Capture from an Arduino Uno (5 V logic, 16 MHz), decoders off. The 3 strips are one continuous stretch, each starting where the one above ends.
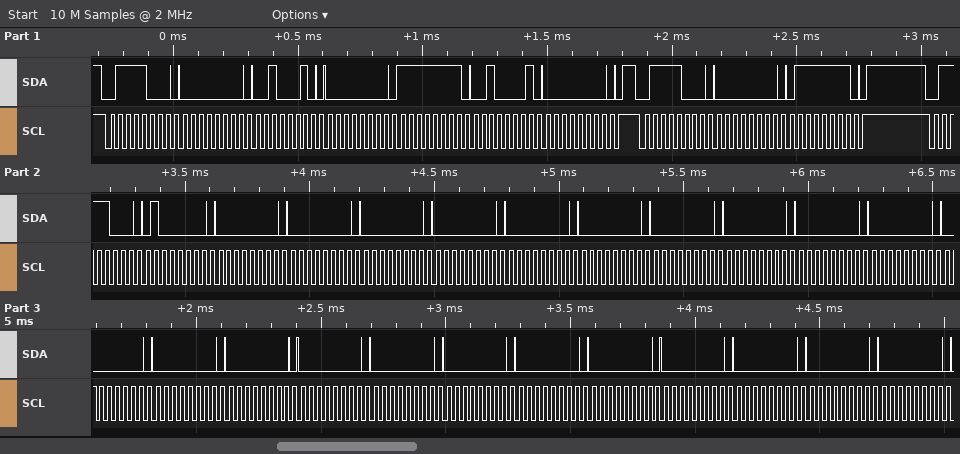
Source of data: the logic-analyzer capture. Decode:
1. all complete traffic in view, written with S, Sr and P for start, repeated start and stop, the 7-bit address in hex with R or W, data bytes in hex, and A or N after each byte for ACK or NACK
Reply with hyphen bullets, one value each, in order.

- S 3CW A 00 A 22 A 00 A FF A 21 A 00 A P S 3CW A 00 A 7F A P S 3CW A 40 A 00 A 00 A 00 A 00 A 00 A 00 A 00 A 00 A 00 A 00 A 00 A 00 A 00 A 00 A 00 A 00 A 00 A 00 A 00 A 00 A 00 A 00 A
